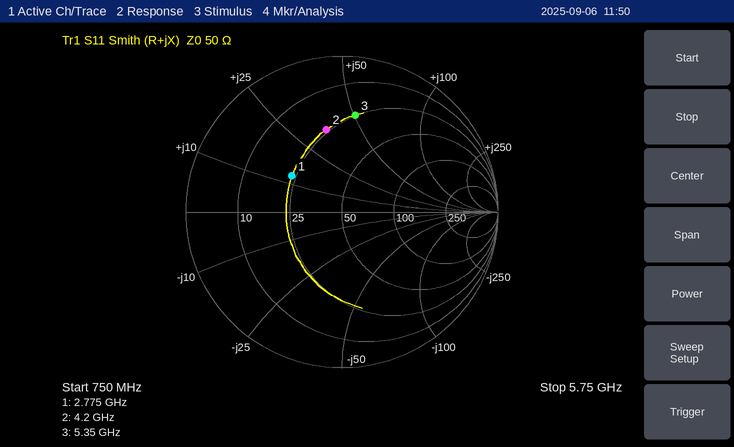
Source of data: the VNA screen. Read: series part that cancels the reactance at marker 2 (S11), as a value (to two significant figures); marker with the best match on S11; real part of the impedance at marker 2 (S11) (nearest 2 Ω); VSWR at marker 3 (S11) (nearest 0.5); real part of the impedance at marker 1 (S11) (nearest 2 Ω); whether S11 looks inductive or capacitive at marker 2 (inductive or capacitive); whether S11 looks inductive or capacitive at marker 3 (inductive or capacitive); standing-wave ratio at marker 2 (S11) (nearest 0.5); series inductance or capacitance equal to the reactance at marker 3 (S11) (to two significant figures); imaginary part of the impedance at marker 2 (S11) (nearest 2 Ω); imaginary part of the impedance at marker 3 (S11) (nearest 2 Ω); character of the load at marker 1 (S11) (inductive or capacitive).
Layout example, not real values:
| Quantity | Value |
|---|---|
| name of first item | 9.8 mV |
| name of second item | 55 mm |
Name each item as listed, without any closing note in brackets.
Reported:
| Quantity | Value |
|---|---|
| series part that cancels the reactance at marker 2 (S11), as a value | 1.1 pF |
| marker with the best match on S11 | marker 1 |
| real part of the impedance at marker 2 (S11) | 24 Ω |
| VSWR at marker 3 (S11) | 4.5 |
| real part of the impedance at marker 1 (S11) | 24 Ω |
| whether S11 looks inductive or capacitive at marker 2 | inductive |
| whether S11 looks inductive or capacitive at marker 3 | inductive |
| standing-wave ratio at marker 2 (S11) | 3.5 |
| series inductance or capacitance equal to the reactance at marker 3 (S11) | 1.5 nH |
| imaginary part of the impedance at marker 2 (S11) | +36 Ω |
| imaginary part of the impedance at marker 3 (S11) | +50 Ω |
| character of the load at marker 1 (S11) | inductive |
